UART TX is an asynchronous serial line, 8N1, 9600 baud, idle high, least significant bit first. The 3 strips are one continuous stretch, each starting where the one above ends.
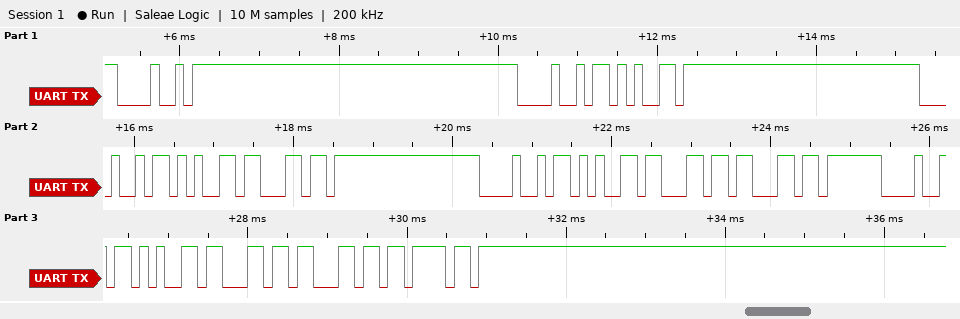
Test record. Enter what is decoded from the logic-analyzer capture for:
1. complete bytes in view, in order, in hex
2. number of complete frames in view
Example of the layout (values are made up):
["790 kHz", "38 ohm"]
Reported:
["0x48 0x48 0x65 0x48 0x65 0x6C 0x48 0x65 0x6C 0x6C 0x48 0x65 0x6C 0x6C 0x6F", "15"]
